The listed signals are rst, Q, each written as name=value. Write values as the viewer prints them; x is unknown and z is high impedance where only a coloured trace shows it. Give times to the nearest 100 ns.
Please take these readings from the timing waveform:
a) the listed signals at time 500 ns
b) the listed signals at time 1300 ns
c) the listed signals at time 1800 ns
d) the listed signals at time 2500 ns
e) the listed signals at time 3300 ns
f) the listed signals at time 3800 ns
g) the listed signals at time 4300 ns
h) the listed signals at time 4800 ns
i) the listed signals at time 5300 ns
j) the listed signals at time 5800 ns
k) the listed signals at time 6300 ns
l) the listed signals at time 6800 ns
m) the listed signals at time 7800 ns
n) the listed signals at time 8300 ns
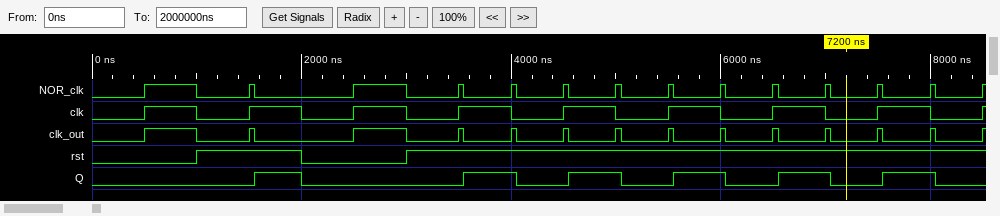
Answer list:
rst=0, Q=0
rst=1, Q=0
rst=1, Q=1
rst=0, Q=0
rst=1, Q=0
rst=1, Q=1
rst=1, Q=0
rst=1, Q=1
rst=1, Q=0
rst=1, Q=1
rst=1, Q=0
rst=1, Q=1
rst=1, Q=1
rst=1, Q=0
